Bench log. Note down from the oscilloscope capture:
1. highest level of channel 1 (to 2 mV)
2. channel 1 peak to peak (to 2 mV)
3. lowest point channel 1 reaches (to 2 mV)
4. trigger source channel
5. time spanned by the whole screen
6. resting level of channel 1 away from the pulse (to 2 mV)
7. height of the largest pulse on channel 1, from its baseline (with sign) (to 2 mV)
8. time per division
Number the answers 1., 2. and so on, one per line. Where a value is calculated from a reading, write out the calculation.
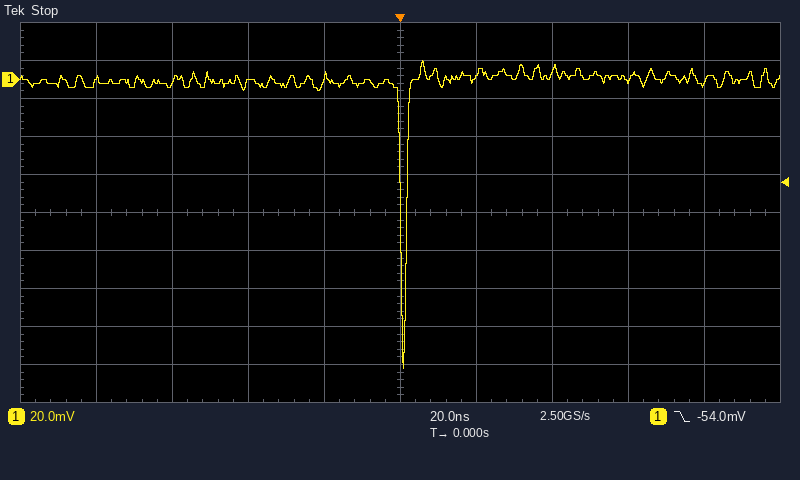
1. 10 mV
2. 10 mV − (-152 mV) = 162 mV
3. -152 mV
4. channel 1
5. 200 ns
6. 0 mV
7. -152 mV − (0 mV) = -152 mV
8. 20 ns
